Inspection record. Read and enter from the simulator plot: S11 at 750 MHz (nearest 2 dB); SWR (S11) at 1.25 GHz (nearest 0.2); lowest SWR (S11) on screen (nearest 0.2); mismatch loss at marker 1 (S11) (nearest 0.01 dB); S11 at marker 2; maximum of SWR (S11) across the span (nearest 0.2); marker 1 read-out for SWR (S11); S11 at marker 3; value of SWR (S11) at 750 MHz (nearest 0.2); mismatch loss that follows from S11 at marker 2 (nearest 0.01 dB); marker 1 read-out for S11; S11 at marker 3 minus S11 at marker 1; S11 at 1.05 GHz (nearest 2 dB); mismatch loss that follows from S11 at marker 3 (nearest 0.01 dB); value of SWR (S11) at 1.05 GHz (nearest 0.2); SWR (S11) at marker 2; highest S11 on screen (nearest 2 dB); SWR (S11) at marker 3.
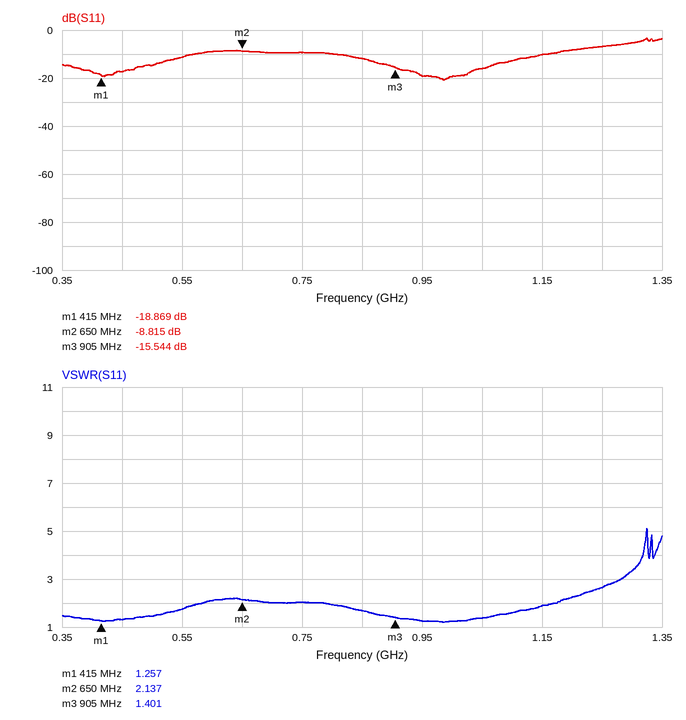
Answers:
-10 dB
2.6
1.2
0.06 dB
-8.815 dB
5.2
1.257
-15.544 dB
2.0
0.61 dB
-18.869 dB
3.325 dB
-16 dB
0.12 dB
1.4
2.137
-4 dB
1.401
